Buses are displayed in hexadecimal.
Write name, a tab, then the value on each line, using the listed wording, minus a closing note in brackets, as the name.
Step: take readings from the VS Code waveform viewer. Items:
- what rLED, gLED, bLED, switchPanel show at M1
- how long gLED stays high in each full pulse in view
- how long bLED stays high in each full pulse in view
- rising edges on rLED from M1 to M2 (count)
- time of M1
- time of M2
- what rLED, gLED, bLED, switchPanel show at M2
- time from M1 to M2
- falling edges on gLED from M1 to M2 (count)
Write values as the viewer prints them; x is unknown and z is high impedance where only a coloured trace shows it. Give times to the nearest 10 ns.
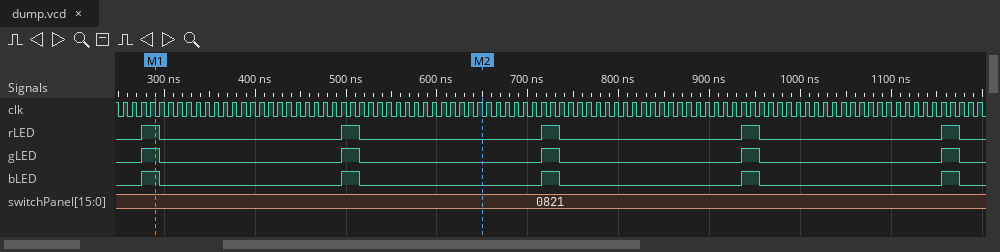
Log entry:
what rLED, gLED, bLED, switchPanel show at M1	rLED=1, gLED=1, bLED=1, switchPanel=0821
how long gLED stays high in each full pulse in view	20 ns, 20 ns, 20 ns, 20 ns, 20 ns
how long bLED stays high in each full pulse in view	20 ns, 20 ns, 20 ns, 20 ns, 20 ns
rising edges on rLED from M1 to M2	1
time of M1	290 ns
time of M2	650 ns
what rLED, gLED, bLED, switchPanel show at M2	rLED=0, gLED=0, bLED=0, switchPanel=0821
time from M1 to M2	360 ns
falling edges on gLED from M1 to M2	2
